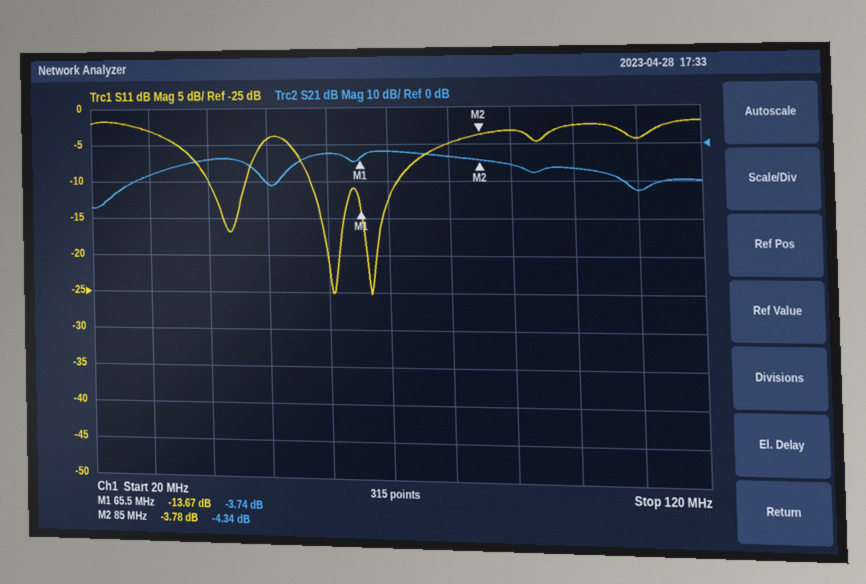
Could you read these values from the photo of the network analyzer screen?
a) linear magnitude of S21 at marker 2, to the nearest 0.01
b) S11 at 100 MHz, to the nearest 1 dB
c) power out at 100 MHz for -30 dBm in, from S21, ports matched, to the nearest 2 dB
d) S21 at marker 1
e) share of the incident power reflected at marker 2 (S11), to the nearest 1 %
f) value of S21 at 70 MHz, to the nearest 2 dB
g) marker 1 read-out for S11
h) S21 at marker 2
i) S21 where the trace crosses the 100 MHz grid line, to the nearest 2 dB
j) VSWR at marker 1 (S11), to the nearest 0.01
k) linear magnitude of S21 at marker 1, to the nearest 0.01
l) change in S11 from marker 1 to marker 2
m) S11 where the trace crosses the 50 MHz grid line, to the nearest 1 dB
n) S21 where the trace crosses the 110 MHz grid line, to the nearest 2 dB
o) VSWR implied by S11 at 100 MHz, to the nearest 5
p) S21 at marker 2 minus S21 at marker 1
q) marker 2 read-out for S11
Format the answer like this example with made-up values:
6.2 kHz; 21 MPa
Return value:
0.61; -3 dB; -36 dBm; -3.74 dB; 42 %; -2 dB; -13.67 dB; -4.34 dB; -6 dB; 1.52; 0.65; 9.89 dB; -4 dB; -12 dB; 5; -0.60 dB; -3.78 dB
